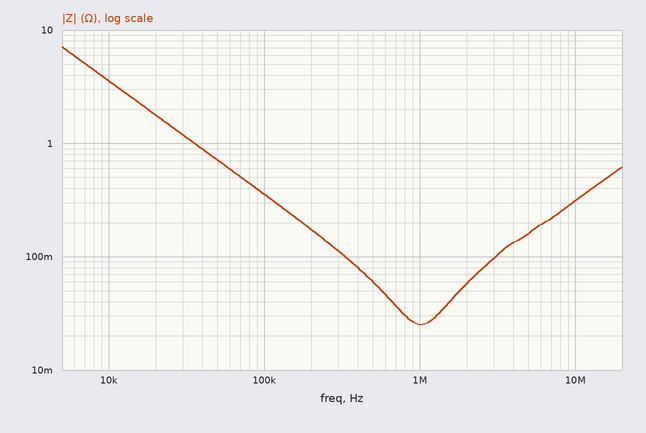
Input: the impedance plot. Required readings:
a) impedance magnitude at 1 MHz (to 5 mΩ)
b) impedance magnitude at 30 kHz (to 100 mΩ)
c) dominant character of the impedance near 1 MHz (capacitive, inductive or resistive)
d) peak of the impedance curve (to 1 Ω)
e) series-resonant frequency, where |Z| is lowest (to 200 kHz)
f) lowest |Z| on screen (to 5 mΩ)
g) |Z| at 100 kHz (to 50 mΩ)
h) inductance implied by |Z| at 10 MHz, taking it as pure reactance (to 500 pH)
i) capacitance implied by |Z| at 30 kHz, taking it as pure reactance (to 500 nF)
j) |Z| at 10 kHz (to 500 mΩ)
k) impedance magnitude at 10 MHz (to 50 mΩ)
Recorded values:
25 mΩ
1.2 Ω
resistive
7 Ω
1.0 MHz
25 mΩ
350 mΩ
5.0 nH
4.5 µF
3.5 Ω
300 mΩ
